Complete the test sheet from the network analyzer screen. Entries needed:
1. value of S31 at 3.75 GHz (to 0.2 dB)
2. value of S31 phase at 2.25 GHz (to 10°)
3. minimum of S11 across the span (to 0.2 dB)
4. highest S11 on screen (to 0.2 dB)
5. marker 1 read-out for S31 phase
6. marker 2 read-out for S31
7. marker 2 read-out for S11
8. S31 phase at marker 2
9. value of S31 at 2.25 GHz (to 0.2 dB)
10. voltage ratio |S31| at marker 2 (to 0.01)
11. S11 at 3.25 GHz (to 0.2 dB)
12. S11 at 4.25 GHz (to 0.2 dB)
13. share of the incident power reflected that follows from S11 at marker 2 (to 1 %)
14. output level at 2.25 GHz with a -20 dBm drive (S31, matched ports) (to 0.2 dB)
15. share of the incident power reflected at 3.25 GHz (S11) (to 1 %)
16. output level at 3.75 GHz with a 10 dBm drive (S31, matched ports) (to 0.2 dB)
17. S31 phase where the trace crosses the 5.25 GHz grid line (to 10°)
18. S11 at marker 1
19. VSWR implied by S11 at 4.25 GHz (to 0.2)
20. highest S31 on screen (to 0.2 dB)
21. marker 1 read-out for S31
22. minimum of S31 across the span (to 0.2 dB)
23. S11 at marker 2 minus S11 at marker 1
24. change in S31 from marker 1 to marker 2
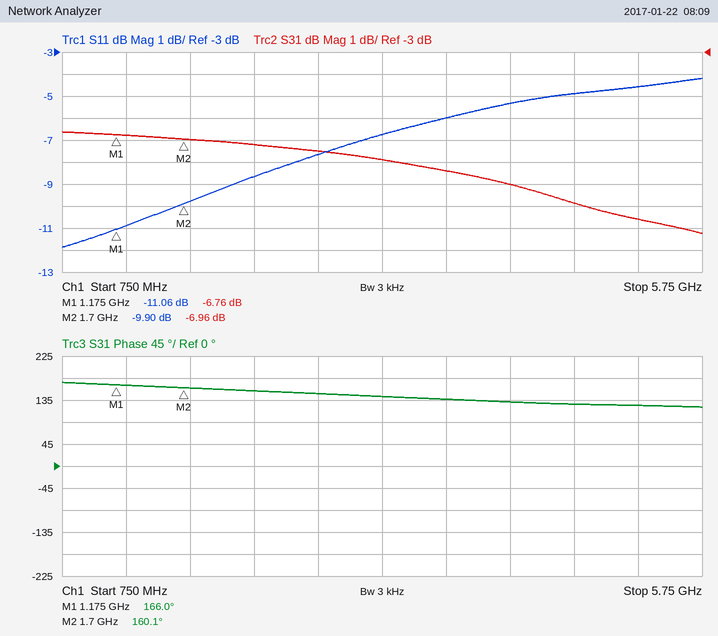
-8.4 dB
150°
-11.8 dB
-4.2 dB
166.0°
-6.96 dB
-9.90 dB
160.1°
-7.2 dB
0.45
-6.8 dB
-5.4 dB
10 %
-27.2 dBm
21 %
1.6 dBm
120°
-11.06 dB
3.4
-6.6 dB
-6.76 dB
-11.2 dB
1.16 dB
-0.20 dB
